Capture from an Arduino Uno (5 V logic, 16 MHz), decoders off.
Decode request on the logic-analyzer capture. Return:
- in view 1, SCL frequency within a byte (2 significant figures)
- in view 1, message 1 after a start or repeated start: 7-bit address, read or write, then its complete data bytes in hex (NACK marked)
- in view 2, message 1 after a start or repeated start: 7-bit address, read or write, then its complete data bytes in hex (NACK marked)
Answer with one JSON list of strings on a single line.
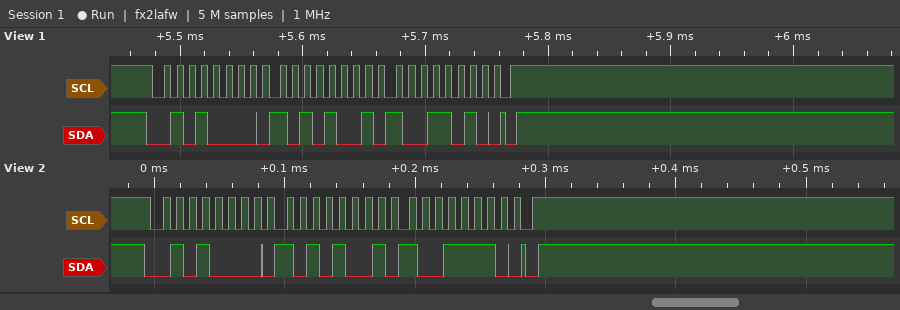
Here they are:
["100 kHz", "0x28 write: A9 9A", "0x28 write: A9 9E"]
